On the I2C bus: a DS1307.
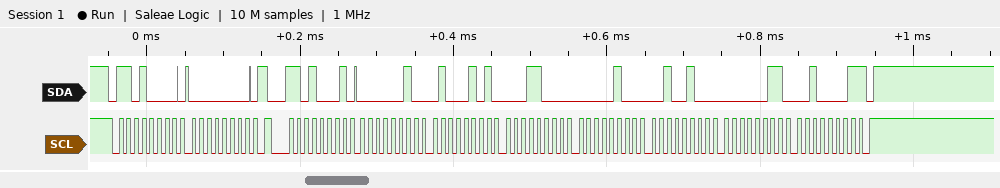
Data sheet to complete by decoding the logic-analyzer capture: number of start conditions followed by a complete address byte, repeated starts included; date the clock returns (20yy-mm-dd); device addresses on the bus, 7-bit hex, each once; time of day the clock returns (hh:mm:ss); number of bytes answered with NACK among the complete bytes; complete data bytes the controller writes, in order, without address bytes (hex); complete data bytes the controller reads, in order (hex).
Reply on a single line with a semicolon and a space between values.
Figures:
2; 2021-03-24; 0x68; 18:45:02; 1; 00; 02 45 18 04 24 03 21
